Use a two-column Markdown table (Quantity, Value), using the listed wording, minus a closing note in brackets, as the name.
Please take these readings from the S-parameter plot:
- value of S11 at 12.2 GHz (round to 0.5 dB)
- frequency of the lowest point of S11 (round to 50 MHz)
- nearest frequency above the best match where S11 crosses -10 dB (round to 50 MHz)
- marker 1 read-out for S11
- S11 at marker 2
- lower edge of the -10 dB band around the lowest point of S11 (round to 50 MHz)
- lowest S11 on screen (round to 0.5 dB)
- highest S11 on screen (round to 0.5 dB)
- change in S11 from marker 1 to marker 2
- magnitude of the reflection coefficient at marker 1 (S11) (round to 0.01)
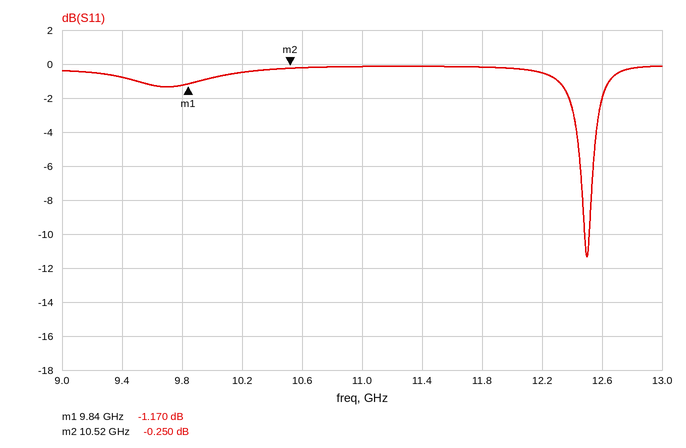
| Quantity | Value |
|---|---|
| value of S11 at 12.2 GHz | -0.5 dB |
| frequency of the lowest point of S11 | 12.50 GHz |
| nearest frequency above the best match where S11 crosses -10 dB | 12.50 GHz |
| marker 1 read-out for S11 | -1.170 dB |
| S11 at marker 2 | -0.250 dB |
| lower edge of the -10 dB band around the lowest point of S11 | 12.50 GHz |
| lowest S11 on screen | -11.5 dB |
| highest S11 on screen | 0.0 dB |
| change in S11 from marker 1 to marker 2 | 0.920 dB |
| magnitude of the reflection coefficient at marker 1 (S11) | 0.87 |
